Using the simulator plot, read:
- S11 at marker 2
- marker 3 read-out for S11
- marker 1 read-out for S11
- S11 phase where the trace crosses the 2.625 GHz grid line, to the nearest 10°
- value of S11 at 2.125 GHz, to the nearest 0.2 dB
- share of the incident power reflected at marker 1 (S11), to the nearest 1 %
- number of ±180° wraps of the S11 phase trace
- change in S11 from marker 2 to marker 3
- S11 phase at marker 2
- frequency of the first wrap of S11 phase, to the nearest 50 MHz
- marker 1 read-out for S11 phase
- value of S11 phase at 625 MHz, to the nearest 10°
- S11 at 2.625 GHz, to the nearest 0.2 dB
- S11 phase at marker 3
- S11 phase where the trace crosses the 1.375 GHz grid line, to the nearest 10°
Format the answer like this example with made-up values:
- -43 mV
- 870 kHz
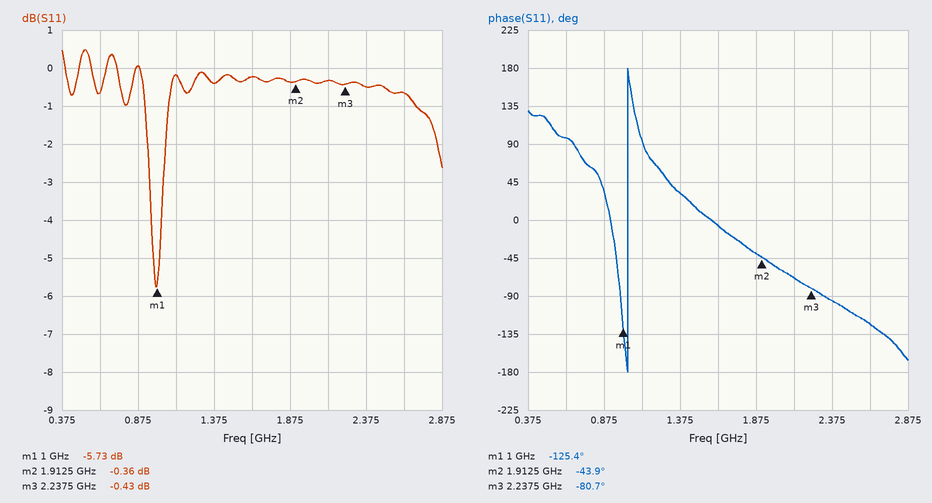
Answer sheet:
- -0.36 dB
- -0.43 dB
- -5.73 dB
- -120°
- -0.4 dB
- 27 %
- 1
- -0.07 dB
- -43.9°
- 1.05 GHz
- -125.4°
- 100°
- -0.6 dB
- -80.7°
- 30°
